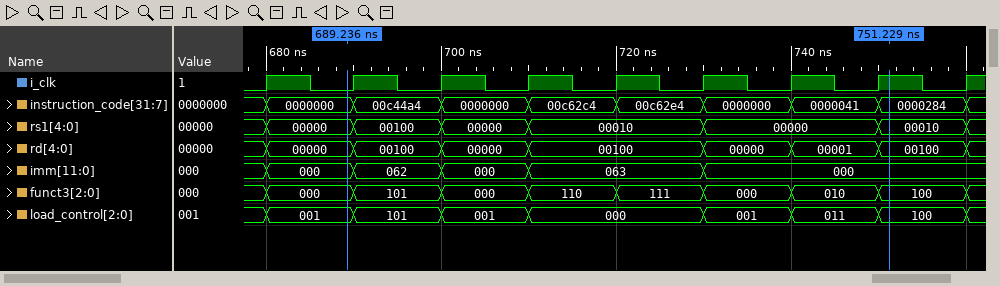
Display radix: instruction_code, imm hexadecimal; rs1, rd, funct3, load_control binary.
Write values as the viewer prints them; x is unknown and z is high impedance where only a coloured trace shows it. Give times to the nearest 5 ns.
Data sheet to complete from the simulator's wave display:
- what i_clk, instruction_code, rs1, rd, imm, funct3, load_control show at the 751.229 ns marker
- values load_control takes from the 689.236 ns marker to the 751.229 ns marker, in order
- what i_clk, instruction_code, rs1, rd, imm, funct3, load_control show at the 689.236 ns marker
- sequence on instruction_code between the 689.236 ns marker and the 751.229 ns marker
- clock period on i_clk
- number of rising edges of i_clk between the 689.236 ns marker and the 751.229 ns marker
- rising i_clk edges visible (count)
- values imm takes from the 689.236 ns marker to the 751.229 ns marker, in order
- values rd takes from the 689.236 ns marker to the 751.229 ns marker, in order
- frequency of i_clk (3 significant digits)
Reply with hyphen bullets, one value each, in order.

- i_clk=1, instruction_code=0000284, rs1=00010, rd=00100, imm=000, funct3=100, load_control=100
- 001, 101, 001, 000, 001, 011, 100
- i_clk=0, instruction_code=0000000, rs1=00000, rd=00000, imm=000, funct3=000, load_control=001
- 0000000, 00c44a4, 0000000, 00c62c4, 00c62e4, 0000000, 0000041, 0000284
- 10 ns
- 7
- 9
- 000, 062, 000, 063, 000
- 00000, 00100, 00000, 00100, 00000, 00001, 00100
- 100 MHz
